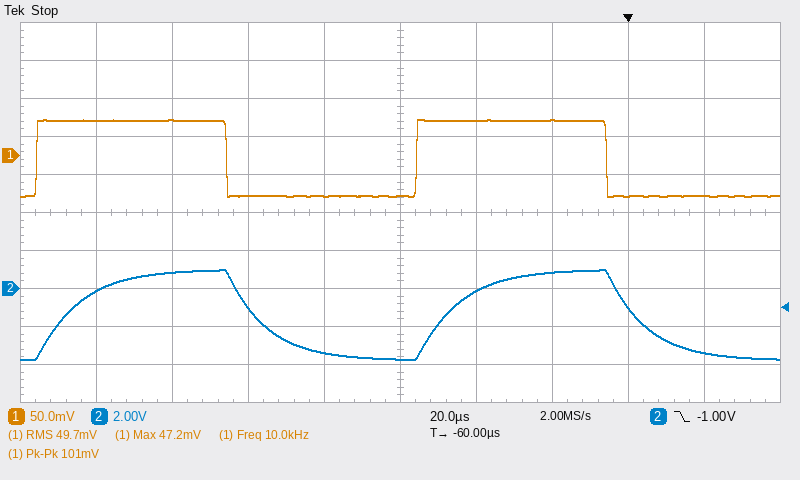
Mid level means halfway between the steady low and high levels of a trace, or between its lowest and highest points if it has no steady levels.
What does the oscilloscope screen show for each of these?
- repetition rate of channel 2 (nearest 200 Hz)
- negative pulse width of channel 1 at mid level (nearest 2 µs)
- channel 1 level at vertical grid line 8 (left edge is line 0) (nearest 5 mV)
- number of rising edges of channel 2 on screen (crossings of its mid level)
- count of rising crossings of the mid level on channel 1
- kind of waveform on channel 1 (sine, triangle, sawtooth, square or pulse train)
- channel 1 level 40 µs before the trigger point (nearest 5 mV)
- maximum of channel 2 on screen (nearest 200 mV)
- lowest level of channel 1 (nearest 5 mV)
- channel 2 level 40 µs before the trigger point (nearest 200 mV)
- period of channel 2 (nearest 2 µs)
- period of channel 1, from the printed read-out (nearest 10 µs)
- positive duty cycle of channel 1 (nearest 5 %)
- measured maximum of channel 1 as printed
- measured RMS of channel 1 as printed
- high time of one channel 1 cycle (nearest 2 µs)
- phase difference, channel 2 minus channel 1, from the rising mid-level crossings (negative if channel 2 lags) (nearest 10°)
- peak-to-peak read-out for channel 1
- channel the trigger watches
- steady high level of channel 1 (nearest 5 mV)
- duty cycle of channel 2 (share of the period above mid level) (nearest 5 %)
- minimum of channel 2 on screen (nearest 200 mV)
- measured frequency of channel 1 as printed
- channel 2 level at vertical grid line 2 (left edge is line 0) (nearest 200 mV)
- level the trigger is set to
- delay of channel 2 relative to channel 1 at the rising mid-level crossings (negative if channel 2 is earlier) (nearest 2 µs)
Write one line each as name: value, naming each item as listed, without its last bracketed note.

repetition rate of channel 2: 10.0 kHz
negative pulse width of channel 1 at mid level: 50 µs
channel 1 level at vertical grid line 8 (left edge is line 0): -55 mV
number of rising edges of channel 2 on screen: 2
count of rising crossings of the mid level on channel 1: 2
kind of waveform on channel 1: square
channel 1 level 40 µs before the trigger point: 45 mV
maximum of channel 2 on screen: 1.0 V
lowest level of channel 1: -55 mV
channel 2 level 40 µs before the trigger point: -200 mV
period of channel 2: 100 µs
period of channel 1, from the printed read-out: 100 µs
positive duty cycle of channel 1: 50 %
measured maximum of channel 1 as printed: 47.2 mV
measured RMS of channel 1 as printed: 49.7 mV
high time of one channel 1 cycle: 50 µs
phase difference, channel 2 minus channel 1, from the rising mid-level crossings (negative if channel 2 lags): -30°
peak-to-peak read-out for channel 1: 101 mV
channel the trigger watches: channel 2
steady high level of channel 1: 45 mV
duty cycle of channel 2 (share of the period above mid level): 50 %
minimum of channel 2 on screen: -3.8 V
measured frequency of channel 1 as printed: 10.0 kHz
channel 2 level at vertical grid line 2 (left edge is line 0): 800 mV
level the trigger is set to: -1.00 V
delay of channel 2 relative to channel 1 at the rising mid-level crossings (negative if channel 2 is earlier): +8 µs
